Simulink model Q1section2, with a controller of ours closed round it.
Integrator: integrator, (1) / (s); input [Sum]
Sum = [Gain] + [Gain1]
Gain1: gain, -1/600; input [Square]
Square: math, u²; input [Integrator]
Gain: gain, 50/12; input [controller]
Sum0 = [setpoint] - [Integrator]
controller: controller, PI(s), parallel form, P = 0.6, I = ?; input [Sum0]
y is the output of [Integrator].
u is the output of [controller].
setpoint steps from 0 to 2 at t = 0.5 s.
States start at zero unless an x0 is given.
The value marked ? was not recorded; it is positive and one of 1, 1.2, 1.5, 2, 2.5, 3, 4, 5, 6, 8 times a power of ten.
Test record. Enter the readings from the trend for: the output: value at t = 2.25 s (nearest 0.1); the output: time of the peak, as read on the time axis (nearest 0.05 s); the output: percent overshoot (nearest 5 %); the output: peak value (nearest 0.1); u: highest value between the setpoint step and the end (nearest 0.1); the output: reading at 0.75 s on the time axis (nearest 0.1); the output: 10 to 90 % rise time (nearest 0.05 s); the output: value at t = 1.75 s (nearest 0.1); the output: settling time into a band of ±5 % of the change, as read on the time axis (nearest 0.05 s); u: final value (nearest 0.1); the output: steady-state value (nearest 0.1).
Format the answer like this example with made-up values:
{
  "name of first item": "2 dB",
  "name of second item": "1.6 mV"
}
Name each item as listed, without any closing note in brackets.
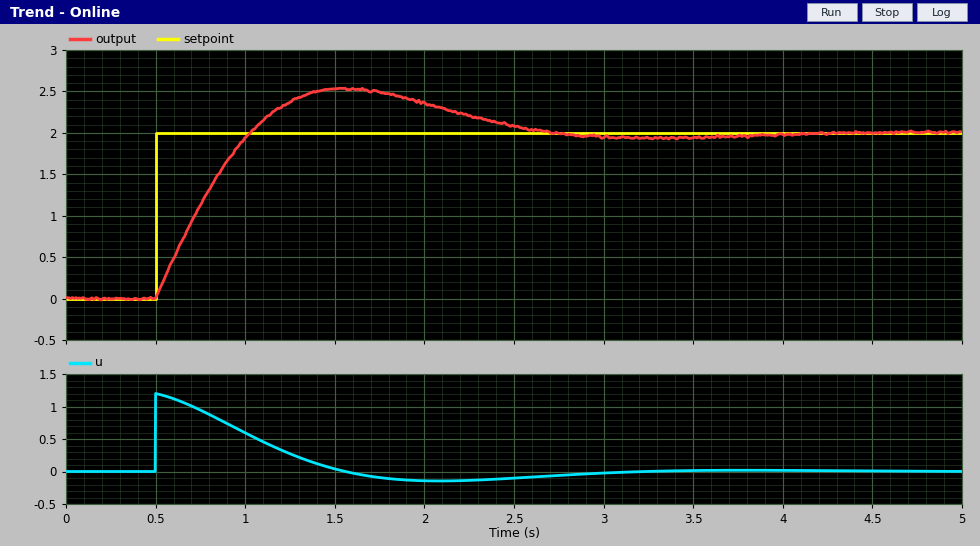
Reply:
{
  "the output: value at t = 2.25 s": "2.2",
  "the output: time of the peak, as read on the time axis": "1.55 s",
  "the output: percent overshoot": "25 %",
  "the output: peak value": "2.5",
  "u: highest value between the setpoint step and the end": "1.2",
  "the output: reading at 0.75 s on the time axis": "1.1",
  "the output: 10 to 90 % rise time": "0.40 s",
  "the output: value at t = 1.75 s": "2.5",
  "the output: settling time into a band of ±5 % of the change, as read on the time axis": "2.45 s",
  "u: final value": "0.0",
  "the output: steady-state value": "2.0"
}
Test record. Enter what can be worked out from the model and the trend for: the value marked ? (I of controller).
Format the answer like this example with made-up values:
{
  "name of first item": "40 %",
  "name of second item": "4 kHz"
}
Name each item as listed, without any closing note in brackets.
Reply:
{
  "the value marked ?": "1.2"
}
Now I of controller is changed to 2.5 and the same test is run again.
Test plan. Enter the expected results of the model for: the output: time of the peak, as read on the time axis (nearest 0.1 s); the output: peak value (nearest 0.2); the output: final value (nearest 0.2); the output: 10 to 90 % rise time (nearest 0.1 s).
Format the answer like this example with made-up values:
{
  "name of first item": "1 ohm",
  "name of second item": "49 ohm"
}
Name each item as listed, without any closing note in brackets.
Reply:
{
  "the output: time of the peak, as read on the time axis": "1.3 s",
  "the output: peak value": "2.8",
  "the output: final value": "2.0",
  "the output: 10 to 90 % rise time": "0.3 s"
}
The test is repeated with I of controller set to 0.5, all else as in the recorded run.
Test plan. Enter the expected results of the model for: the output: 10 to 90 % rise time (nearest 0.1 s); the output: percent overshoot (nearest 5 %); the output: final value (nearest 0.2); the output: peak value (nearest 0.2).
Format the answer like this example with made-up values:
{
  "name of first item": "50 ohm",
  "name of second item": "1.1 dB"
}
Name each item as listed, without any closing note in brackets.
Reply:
{
  "the output: 10 to 90 % rise time": "0.5 s",
  "the output: percent overshoot": "15 %",
  "the output: final value": "2.0",
  "the output: peak value": "2.4"
}
